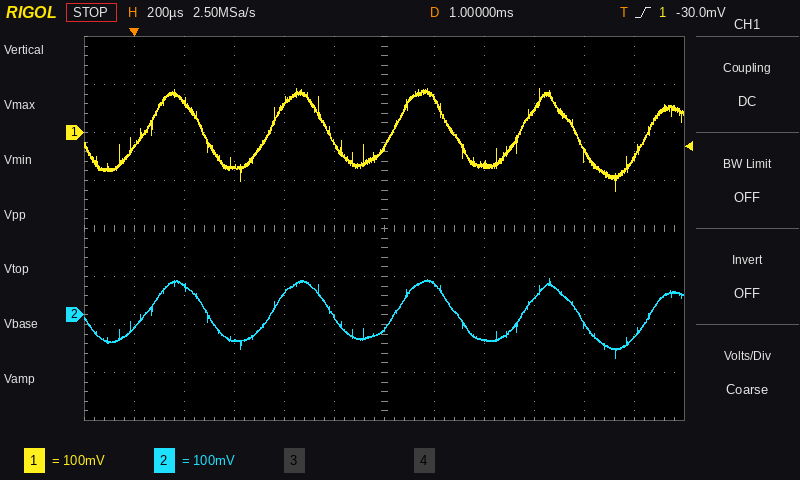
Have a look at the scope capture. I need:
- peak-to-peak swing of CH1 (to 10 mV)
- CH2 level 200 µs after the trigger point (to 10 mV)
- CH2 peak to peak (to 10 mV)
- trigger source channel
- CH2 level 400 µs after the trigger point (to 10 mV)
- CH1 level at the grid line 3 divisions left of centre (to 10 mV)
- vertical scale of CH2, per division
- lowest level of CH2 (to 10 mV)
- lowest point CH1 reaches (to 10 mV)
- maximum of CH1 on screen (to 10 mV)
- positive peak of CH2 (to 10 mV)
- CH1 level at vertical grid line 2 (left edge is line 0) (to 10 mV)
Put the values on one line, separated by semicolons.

210 mV; 60 mV; 170 mV; CH1; -50 mV; -70 mV; 100 mV; -90 mV; -120 mV; 90 mV; 80 mV; 60 mV
